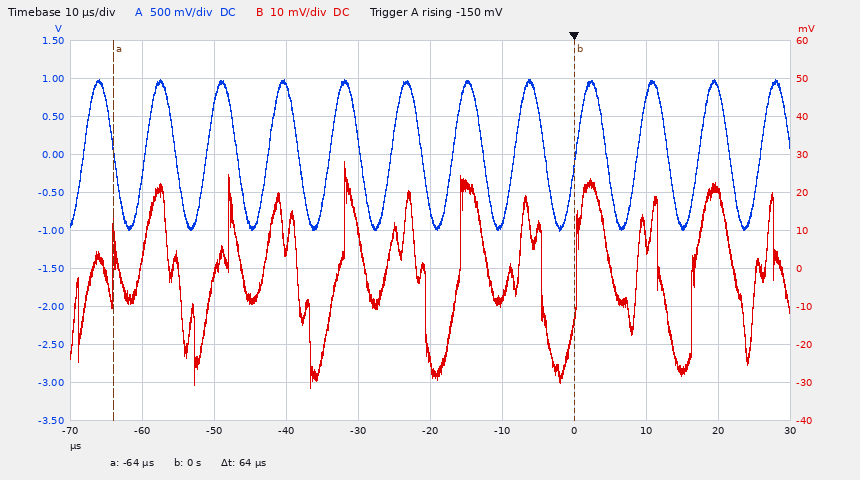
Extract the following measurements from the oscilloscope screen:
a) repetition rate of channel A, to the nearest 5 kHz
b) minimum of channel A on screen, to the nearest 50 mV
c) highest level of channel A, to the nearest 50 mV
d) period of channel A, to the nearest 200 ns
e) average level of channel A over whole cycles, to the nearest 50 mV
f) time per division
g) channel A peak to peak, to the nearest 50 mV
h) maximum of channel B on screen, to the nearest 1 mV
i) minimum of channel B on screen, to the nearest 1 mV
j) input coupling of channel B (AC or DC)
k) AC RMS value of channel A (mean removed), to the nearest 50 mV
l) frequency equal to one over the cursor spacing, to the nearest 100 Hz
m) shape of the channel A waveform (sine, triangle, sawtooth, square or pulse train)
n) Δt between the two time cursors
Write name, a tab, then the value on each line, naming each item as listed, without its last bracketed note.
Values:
repetition rate of channel A, to the nearest 5 kHz	115 kHz
minimum of channel A on screen, to the nearest 50 mV	-1.00 V
highest level of channel A, to the nearest 50 mV	1.00 V
period of channel A, to the nearest 200 ns	8.6 µs
average level of channel A over whole cycles, to the nearest 50 mV	0 mV
time per division	10 µs
channel A peak to peak, to the nearest 50 mV	2.00 V
maximum of channel B on screen, to the nearest 1 mV	28 mV
minimum of channel B on screen, to the nearest 1 mV	-31 mV
input coupling of channel B	DC
AC RMS value of channel A (mean removed), to the nearest 50 mV	700 mV
frequency equal to one over the cursor spacing, to the nearest 100 Hz	15.6 kHz
shape of the channel A waveform	sine
Δt between the two time cursors	64 µs
